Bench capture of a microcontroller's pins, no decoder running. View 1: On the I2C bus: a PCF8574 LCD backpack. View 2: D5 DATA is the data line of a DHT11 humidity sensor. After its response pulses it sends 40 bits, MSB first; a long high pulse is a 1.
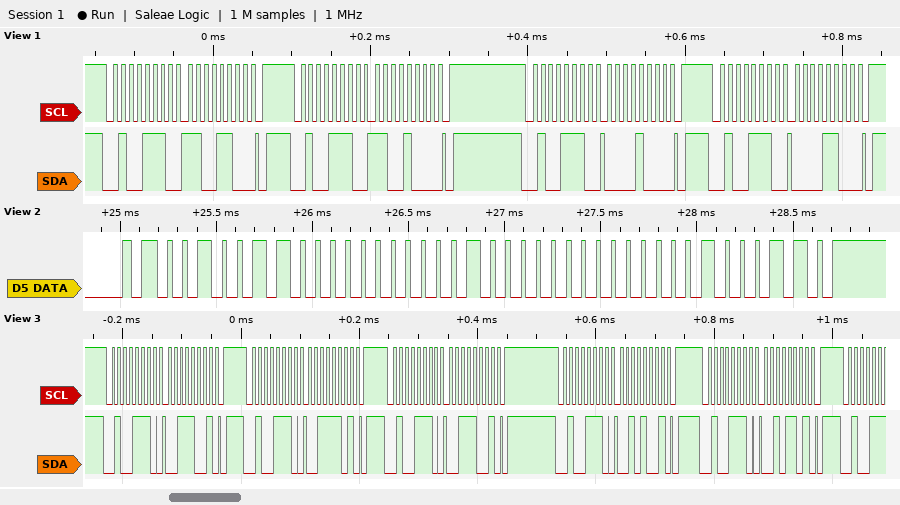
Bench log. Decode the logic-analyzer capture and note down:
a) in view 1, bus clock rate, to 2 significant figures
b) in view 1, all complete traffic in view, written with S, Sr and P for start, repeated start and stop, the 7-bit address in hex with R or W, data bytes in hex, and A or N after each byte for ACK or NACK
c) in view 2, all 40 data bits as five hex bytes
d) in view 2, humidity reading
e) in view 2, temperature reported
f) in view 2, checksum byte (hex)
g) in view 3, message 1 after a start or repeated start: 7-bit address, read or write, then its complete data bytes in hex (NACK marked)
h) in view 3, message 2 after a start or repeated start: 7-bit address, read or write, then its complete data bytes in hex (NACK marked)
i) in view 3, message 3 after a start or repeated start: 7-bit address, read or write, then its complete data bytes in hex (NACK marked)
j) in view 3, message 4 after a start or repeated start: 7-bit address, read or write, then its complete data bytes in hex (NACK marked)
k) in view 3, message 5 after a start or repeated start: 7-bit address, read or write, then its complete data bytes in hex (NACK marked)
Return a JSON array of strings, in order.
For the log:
["100 kHz", "S 27W A CC A P S 27W A C8 A P S 27W A 08 A P S 27W A 0C A P", "26 00 20 00 46", "38 %", "32.0 °C", "0x46", "0x27 write: 39", "0x27 write: 3D", "0x27 write: 39", "0x27 write: 29", "0x27 write: 2D"]
